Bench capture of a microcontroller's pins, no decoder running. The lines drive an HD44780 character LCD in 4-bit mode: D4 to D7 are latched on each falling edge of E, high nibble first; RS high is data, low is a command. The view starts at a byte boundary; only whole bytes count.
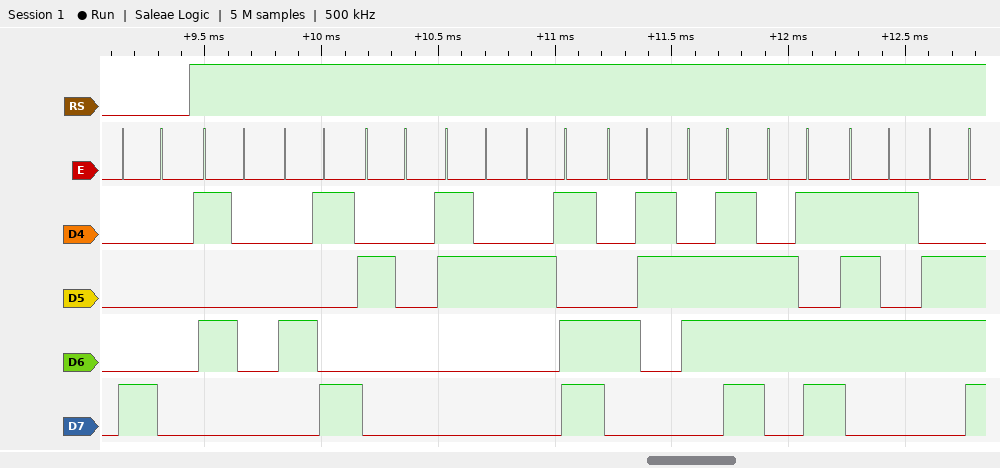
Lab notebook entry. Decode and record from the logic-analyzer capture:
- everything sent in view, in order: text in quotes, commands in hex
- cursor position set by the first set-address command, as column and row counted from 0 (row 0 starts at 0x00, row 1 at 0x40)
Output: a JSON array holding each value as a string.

["0x80 \"PI 2-Comun\"", "column 0, row 0"]
